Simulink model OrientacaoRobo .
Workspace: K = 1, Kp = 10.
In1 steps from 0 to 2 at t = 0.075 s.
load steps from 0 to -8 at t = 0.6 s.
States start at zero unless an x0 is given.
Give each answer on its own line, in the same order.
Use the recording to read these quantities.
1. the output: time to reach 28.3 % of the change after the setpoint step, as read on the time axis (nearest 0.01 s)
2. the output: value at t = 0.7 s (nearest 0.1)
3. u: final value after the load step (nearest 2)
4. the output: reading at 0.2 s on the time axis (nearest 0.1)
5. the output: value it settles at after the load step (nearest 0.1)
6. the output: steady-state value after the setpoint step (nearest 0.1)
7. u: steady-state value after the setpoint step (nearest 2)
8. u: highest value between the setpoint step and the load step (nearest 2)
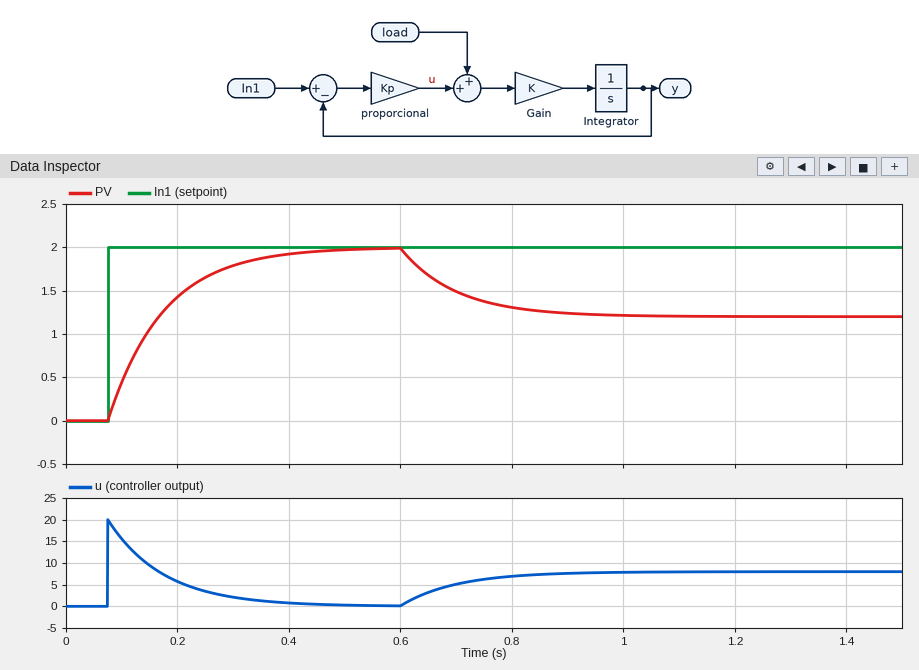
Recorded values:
0.11 s
1.5
8
1.4
1.2
2.0
0
20
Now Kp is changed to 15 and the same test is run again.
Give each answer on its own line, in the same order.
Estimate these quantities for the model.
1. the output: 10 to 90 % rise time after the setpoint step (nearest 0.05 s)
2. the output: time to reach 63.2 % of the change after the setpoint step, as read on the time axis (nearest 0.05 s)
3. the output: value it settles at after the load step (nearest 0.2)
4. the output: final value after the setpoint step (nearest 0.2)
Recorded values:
0.15 s
0.15 s
1.4
2.0
